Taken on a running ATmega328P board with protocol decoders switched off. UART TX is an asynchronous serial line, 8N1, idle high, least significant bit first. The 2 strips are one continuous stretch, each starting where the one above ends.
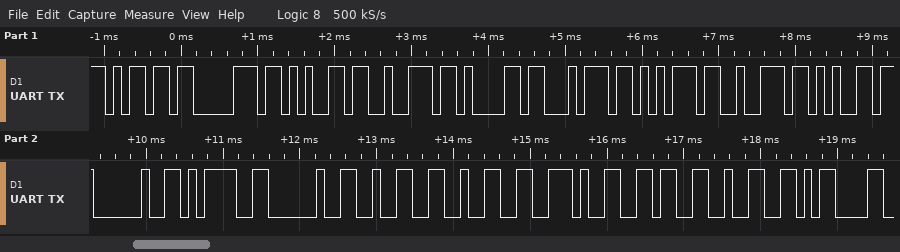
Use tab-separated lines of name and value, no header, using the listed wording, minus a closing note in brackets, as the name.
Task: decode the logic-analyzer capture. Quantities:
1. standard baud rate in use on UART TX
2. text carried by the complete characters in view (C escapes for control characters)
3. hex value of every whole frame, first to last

standard baud rate in use on UART TX	9600 baud
text carried by the complete characters in view	"mperature = 22.62\r"
hex value of every whole frame, first to last	6D 70 65 72 61 74 75 72 65 20 3D 20 32 32 2E 36 32 0D
